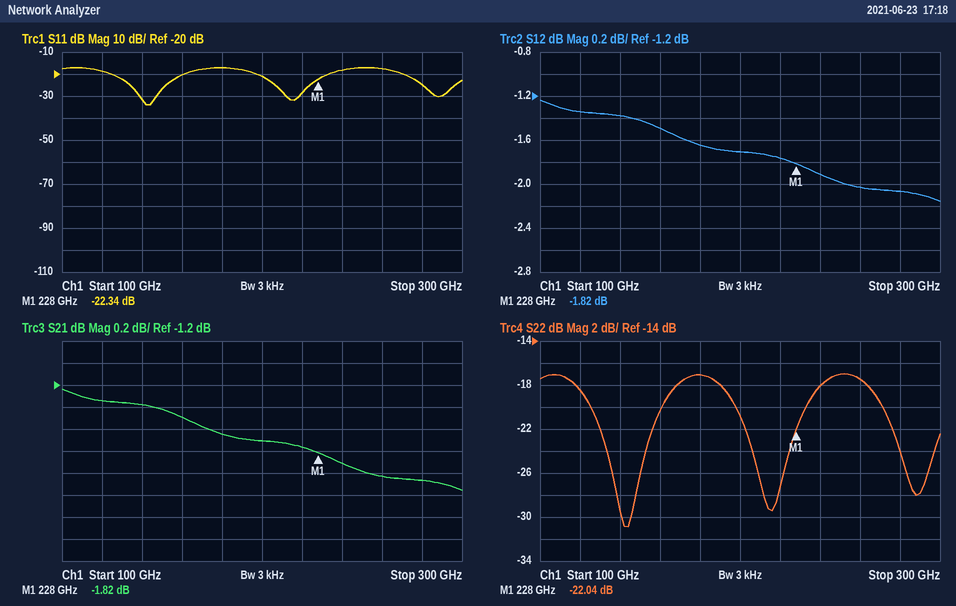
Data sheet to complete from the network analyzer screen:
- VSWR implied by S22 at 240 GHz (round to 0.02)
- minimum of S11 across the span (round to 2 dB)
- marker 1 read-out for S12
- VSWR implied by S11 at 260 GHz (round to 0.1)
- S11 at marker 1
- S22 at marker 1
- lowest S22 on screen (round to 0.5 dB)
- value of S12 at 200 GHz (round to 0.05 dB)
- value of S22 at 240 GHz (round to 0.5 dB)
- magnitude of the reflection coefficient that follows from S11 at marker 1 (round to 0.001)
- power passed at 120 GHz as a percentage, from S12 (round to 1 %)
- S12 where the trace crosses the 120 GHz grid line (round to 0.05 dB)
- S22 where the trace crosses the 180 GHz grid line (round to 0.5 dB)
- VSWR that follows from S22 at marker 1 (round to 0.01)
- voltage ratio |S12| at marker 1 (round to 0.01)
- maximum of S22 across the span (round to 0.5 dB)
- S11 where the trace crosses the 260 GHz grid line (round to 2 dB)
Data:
1.28
-34 dB
-1.82 dB
1.3
-22.34 dB
-22.04 dB
-31.0 dB
-1.70 dB
-18.0 dB
0.076
73 %
-1.35 dB
-17.0 dB
1.17
0.81
-17.0 dB
-18 dB
